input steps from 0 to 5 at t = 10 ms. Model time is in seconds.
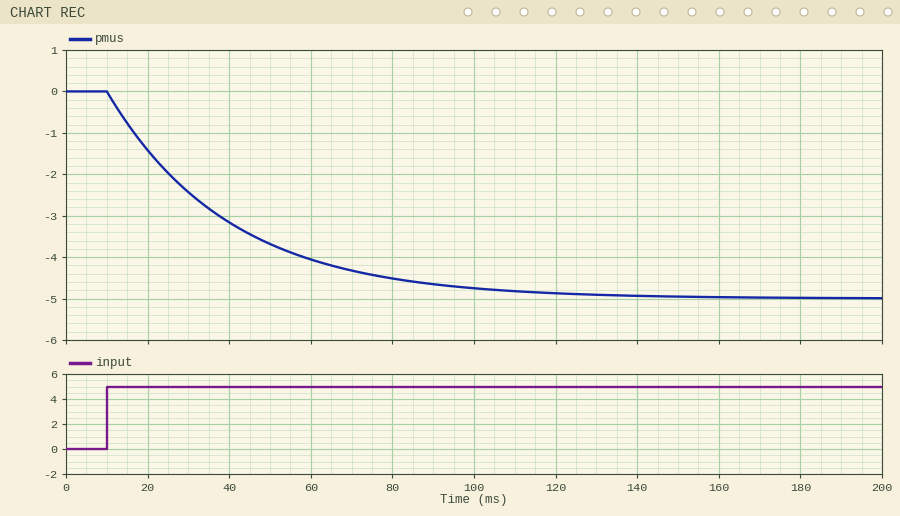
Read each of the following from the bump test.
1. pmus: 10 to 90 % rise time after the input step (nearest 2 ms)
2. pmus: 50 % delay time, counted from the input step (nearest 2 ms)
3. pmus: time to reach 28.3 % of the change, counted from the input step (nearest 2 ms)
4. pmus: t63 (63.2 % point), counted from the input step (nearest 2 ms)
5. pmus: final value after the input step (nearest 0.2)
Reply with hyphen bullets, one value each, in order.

- 66 ms
- 20 ms
- 10 ms
- 30 ms
- -5.0
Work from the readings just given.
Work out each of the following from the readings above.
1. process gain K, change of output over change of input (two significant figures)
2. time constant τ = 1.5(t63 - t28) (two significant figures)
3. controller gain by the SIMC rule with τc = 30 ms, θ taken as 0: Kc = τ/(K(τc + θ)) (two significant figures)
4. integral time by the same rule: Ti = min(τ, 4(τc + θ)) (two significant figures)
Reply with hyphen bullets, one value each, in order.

- -1.0
- 30 ms
- -1.0
- 30 ms
